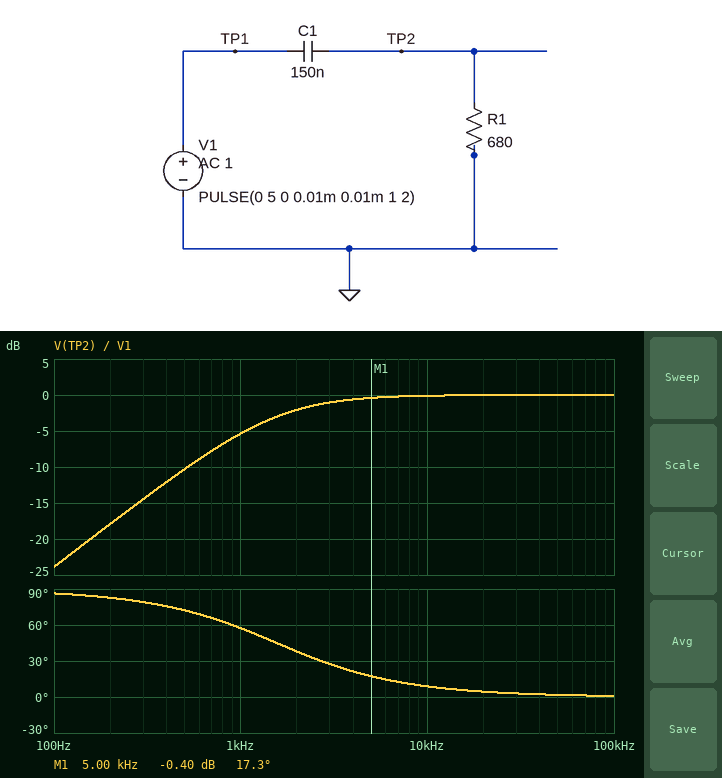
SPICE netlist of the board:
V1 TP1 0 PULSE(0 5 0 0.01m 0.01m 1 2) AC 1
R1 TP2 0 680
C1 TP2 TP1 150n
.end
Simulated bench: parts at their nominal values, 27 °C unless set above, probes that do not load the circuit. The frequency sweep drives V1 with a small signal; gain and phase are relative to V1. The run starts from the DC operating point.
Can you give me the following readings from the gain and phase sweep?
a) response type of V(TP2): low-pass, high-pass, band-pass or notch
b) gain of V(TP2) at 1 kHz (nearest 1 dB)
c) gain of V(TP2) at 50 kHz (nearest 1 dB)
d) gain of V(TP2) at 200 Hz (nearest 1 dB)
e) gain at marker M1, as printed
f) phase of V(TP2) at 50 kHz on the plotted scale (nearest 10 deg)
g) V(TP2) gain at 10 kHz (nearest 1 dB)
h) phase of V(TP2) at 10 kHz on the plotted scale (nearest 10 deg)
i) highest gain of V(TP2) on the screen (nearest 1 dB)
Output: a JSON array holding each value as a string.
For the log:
["high-pass", "-5 dB", "0 dB", "-18 dB", "-0.40 dB", "0 deg", "0 dB", "10 deg", "0 dB"]
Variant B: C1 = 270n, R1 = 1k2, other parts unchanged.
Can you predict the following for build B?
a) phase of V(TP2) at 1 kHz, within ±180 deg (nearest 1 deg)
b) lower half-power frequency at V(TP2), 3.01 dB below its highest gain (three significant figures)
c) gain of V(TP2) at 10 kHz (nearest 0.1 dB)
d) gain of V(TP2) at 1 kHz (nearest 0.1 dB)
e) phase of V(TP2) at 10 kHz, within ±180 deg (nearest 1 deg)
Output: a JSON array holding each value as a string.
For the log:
["26 deg", "491 Hz", "0 dB", "-0.9 dB", "3 deg"]
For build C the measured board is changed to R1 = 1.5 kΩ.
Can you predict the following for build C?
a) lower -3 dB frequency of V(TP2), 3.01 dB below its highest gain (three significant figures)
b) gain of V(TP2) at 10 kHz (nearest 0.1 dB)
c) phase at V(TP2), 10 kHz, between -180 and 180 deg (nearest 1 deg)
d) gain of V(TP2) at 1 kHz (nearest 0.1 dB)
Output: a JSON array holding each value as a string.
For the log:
["707 Hz", "0 dB", "4 deg", "-1.8 dB"]
